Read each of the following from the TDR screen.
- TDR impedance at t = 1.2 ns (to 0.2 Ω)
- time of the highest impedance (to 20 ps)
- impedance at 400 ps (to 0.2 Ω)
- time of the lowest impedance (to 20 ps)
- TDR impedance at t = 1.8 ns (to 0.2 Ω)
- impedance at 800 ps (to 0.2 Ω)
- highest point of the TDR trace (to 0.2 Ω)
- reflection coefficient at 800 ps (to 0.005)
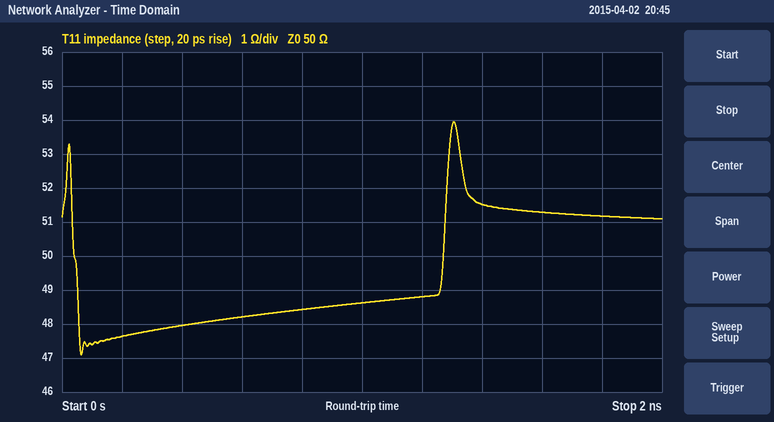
48.8 Ω
1.30 ns
48.0 Ω
60 ps
51.2 Ω
48.4 Ω
54.0 Ω
-0.015
